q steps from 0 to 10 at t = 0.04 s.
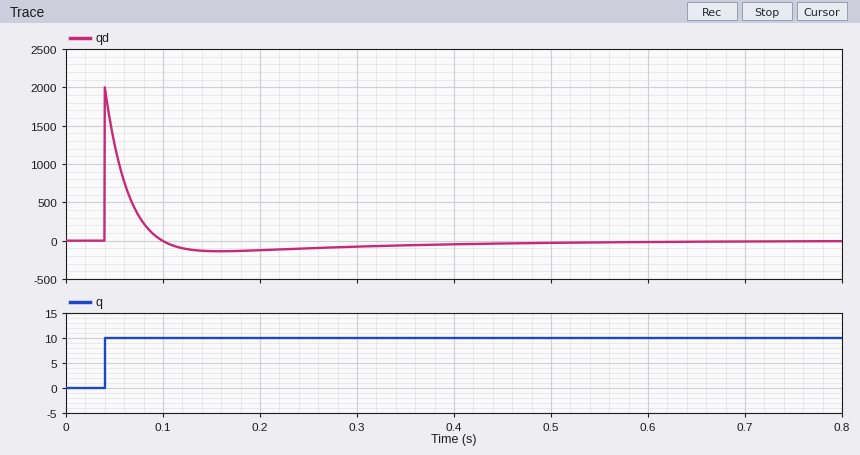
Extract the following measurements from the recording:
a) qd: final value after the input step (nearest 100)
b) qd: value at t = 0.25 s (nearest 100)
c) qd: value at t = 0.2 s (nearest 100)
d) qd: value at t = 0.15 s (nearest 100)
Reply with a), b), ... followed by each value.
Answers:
a) 0
b) -100
c) -100
d) -100
